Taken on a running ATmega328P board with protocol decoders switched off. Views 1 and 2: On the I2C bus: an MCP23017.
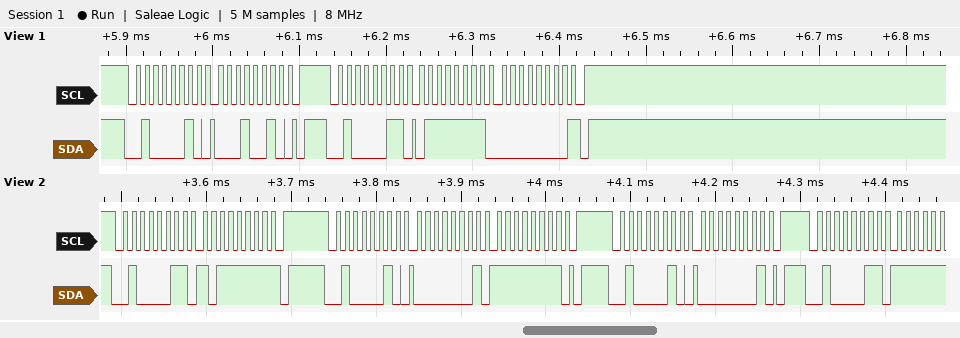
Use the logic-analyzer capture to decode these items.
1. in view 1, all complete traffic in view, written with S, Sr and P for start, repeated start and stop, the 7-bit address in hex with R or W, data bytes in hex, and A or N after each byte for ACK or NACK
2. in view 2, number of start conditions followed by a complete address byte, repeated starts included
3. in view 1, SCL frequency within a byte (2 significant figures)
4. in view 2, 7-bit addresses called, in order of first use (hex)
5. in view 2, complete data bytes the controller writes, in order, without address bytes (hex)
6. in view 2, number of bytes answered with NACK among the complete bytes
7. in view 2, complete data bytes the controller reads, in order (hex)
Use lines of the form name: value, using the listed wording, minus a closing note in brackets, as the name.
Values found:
in view 1, all complete traffic in view, written with S, Sr and P for start, repeated start and stop, the 7-bit address in hex with R or W, data bytes in hex, and A or N after each byte for ACK or NACK: S 21W A 12 A P S 21R A 7F A 00 N P
in view 2, number of start conditions followed by a complete address byte, repeated starts included: 4
in view 1, SCL frequency within a byte: 100 kHz
in view 2, 7-bit addresses called, in order of first use: 0x21
in view 2, complete data bytes the controller writes, in order, without address bytes: 01 FF 01
in view 2, number of bytes answered with NACK among the complete bytes: 1
in view 2, complete data bytes the controller reads, in order: BF
